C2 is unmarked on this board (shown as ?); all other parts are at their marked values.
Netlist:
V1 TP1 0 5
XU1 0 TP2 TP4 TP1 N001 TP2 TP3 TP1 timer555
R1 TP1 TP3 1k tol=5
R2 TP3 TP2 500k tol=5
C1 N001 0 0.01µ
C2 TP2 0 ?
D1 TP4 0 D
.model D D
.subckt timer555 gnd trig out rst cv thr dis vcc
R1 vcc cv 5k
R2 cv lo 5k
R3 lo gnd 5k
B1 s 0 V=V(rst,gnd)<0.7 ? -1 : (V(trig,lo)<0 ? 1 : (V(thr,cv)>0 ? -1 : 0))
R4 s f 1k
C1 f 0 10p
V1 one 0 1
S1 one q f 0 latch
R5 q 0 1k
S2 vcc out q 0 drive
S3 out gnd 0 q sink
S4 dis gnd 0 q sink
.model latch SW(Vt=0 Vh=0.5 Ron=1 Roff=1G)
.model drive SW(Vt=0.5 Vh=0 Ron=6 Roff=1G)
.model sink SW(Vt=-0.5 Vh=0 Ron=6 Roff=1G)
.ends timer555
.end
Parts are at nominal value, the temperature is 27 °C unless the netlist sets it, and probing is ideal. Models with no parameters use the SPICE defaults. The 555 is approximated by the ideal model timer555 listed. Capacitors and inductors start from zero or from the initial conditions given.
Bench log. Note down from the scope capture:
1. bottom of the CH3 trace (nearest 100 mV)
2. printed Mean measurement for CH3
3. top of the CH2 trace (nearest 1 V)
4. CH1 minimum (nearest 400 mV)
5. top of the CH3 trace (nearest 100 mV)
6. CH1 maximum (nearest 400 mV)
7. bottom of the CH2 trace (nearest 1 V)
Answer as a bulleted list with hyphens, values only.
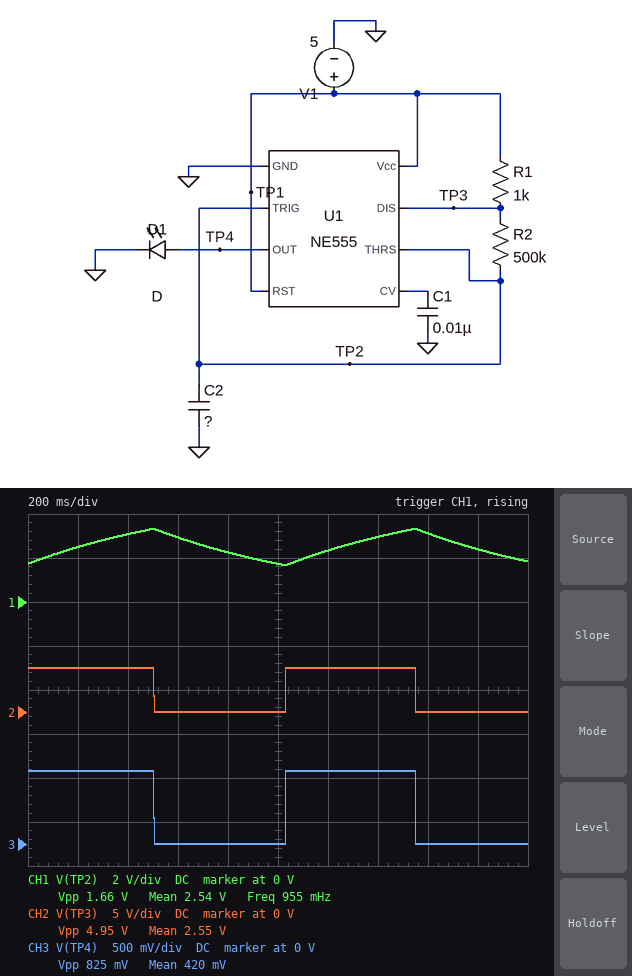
- 0 V
- 420 mV
- 5 V
- 1.6 V
- 800 mV
- 3.2 V
- 0 V
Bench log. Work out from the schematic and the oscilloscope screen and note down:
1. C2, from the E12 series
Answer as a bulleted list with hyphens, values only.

- 1.5 µF
